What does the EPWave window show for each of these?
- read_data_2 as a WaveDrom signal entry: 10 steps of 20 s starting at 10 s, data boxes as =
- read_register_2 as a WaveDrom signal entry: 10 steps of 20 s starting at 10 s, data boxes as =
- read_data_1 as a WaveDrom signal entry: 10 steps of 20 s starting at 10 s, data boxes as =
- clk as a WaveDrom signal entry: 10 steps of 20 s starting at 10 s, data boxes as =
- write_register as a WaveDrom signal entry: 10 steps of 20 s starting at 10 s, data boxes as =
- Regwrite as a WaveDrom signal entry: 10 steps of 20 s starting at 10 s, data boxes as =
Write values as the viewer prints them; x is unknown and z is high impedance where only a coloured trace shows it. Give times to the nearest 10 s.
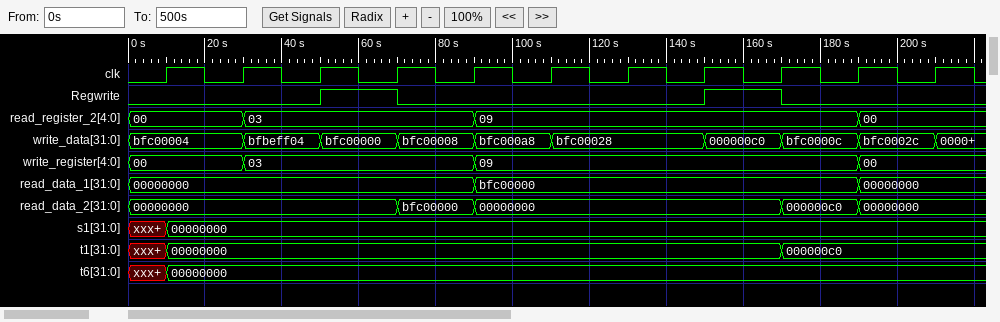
{name: 'read_data_2', wave: '=..==...==', data: '00000000 bfc00000 00000000 000000c0 00000000'}
{name: 'read_register_2', wave: '==..=....=', data: '00 03 09 00'}
{name: 'read_data_1', wave: '=...=....=', data: '00000000 bfc00000 00000000'}
{name: 'clk', wave: 'p.........'}
{name: 'write_register', wave: '==..=....=', data: '00 03 09 00'}
{name: 'Regwrite', wave: '0.10...10.'}
